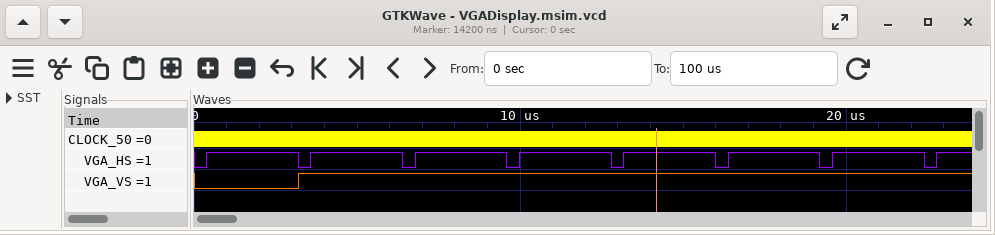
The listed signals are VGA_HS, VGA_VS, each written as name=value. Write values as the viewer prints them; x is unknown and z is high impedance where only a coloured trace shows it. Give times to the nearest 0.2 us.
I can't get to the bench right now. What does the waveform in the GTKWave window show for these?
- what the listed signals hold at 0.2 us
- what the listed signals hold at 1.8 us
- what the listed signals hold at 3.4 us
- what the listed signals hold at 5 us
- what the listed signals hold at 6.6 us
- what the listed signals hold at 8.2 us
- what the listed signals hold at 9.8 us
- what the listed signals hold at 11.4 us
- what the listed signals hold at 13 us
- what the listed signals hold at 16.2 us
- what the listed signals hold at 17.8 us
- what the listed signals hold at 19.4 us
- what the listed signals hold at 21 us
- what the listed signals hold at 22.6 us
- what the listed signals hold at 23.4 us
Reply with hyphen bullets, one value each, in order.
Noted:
- VGA_HS=0, VGA_VS=0
- VGA_HS=1, VGA_VS=0
- VGA_HS=0, VGA_VS=1
- VGA_HS=1, VGA_VS=1
- VGA_HS=0, VGA_VS=1
- VGA_HS=1, VGA_VS=1
- VGA_HS=0, VGA_VS=1
- VGA_HS=1, VGA_VS=1
- VGA_HS=0, VGA_VS=1
- VGA_HS=0, VGA_VS=1
- VGA_HS=1, VGA_VS=1
- VGA_HS=0, VGA_VS=1
- VGA_HS=1, VGA_VS=1
- VGA_HS=0, VGA_VS=1
- VGA_HS=1, VGA_VS=1
